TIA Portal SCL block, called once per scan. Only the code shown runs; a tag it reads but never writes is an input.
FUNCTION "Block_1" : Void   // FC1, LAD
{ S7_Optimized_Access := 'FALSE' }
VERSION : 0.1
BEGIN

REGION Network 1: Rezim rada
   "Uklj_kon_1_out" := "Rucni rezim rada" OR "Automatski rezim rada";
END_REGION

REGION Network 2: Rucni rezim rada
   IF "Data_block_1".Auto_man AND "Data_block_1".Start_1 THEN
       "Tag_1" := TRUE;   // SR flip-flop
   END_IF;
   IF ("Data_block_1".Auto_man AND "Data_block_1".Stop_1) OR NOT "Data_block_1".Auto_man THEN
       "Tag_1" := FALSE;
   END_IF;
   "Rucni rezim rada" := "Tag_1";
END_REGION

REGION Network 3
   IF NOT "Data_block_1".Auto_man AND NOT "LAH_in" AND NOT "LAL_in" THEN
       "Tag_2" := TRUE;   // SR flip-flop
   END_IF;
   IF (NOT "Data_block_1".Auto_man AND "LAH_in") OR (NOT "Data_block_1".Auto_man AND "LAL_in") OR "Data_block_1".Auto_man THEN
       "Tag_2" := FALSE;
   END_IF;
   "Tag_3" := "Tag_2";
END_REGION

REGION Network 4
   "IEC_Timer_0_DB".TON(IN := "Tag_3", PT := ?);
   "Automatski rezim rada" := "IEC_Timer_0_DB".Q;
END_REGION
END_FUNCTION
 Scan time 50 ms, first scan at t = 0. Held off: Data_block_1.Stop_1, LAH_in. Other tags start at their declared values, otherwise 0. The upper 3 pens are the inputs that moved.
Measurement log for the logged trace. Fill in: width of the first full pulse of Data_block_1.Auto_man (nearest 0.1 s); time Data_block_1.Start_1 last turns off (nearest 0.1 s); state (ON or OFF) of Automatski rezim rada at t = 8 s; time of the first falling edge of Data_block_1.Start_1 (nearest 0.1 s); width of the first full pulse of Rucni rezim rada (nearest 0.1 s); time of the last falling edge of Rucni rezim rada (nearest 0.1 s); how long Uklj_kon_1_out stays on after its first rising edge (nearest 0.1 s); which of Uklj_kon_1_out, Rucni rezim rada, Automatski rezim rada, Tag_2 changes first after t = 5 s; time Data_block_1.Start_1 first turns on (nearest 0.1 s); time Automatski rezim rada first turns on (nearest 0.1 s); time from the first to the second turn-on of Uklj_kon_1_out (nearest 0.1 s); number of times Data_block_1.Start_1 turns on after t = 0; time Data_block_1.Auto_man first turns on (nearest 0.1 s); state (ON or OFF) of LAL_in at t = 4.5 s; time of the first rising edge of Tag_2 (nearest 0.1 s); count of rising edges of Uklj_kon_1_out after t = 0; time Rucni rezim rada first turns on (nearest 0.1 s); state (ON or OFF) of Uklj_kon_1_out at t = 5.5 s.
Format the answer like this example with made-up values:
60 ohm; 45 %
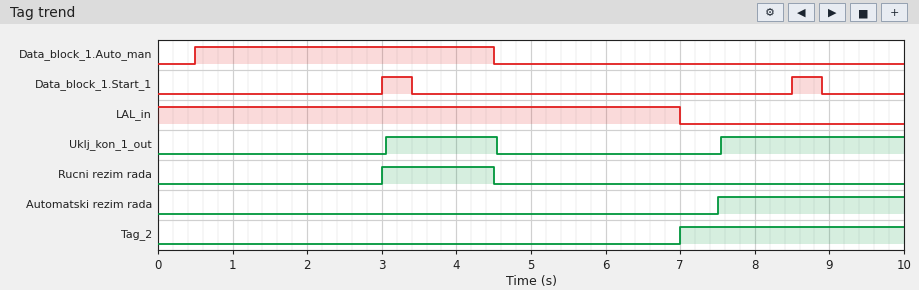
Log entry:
4.0 s; 8.9 s; ON; 3.4 s; 1.5 s; 4.5 s; 1.5 s; Tag_2; 3.0 s; 7.5 s; 4.5 s; 2; 0.5 s; ON; 7.0 s; 2; 3.0 s; OFF
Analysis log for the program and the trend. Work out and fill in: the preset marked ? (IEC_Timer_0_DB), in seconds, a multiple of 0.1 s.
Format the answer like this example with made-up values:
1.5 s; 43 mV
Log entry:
0.5 s
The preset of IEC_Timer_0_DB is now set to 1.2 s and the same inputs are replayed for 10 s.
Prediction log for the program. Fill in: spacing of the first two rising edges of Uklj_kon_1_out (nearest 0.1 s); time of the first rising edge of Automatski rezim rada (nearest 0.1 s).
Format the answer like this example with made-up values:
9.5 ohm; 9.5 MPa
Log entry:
5.2 s; 8.2 s
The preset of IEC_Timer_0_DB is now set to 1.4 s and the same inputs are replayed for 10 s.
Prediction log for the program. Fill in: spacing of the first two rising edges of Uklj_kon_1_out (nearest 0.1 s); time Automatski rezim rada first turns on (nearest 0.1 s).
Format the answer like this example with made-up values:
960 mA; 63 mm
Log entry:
5.4 s; 8.4 s
